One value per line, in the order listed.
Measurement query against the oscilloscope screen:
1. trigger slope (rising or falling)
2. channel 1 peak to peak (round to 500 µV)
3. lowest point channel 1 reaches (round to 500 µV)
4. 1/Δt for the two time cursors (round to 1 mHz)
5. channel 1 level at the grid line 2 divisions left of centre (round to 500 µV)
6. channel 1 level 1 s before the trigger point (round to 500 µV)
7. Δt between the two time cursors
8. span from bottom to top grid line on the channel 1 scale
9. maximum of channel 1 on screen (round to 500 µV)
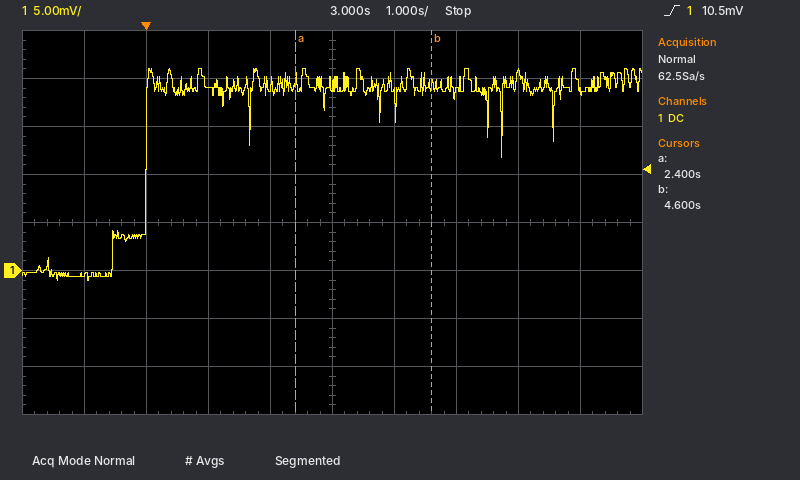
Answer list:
rising
22.0 mV
-1.0 mV
455 mHz
19.0 mV
-500 µV
2.2 s
40 mV
21.0 mV
